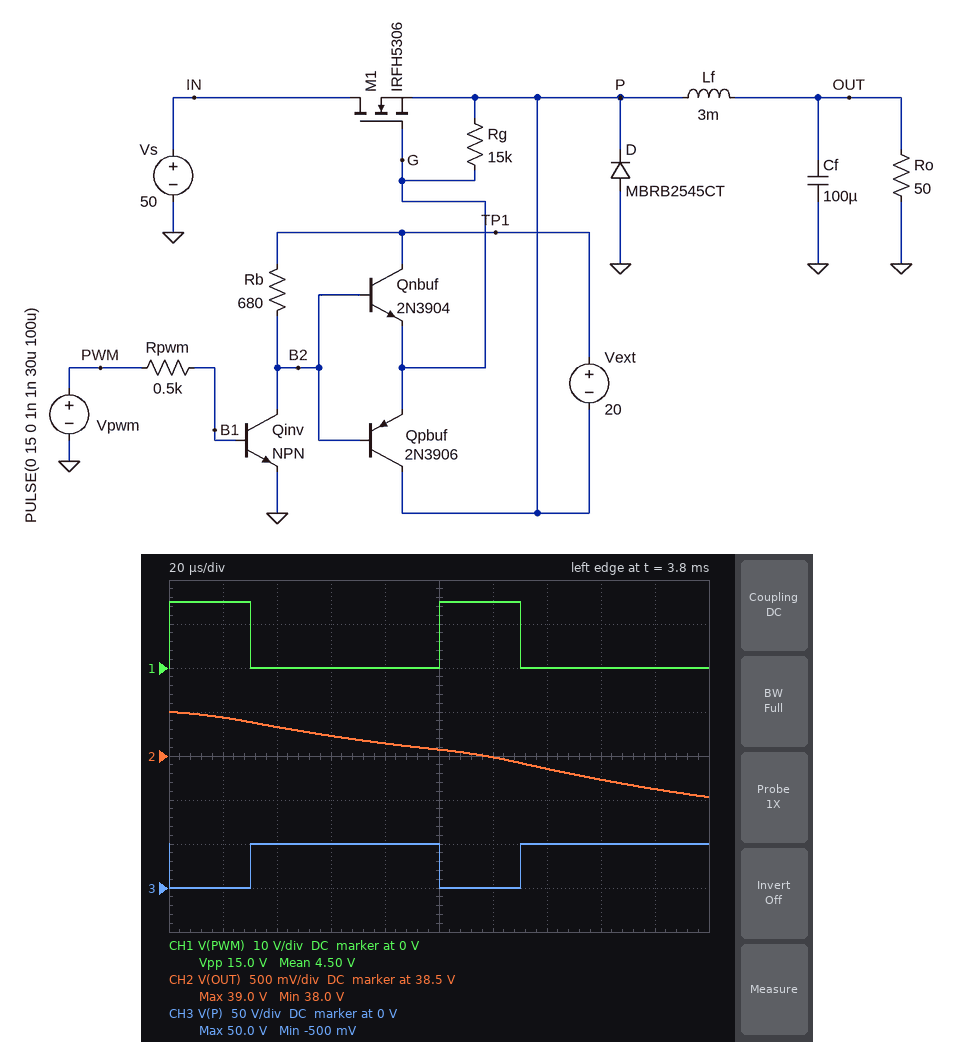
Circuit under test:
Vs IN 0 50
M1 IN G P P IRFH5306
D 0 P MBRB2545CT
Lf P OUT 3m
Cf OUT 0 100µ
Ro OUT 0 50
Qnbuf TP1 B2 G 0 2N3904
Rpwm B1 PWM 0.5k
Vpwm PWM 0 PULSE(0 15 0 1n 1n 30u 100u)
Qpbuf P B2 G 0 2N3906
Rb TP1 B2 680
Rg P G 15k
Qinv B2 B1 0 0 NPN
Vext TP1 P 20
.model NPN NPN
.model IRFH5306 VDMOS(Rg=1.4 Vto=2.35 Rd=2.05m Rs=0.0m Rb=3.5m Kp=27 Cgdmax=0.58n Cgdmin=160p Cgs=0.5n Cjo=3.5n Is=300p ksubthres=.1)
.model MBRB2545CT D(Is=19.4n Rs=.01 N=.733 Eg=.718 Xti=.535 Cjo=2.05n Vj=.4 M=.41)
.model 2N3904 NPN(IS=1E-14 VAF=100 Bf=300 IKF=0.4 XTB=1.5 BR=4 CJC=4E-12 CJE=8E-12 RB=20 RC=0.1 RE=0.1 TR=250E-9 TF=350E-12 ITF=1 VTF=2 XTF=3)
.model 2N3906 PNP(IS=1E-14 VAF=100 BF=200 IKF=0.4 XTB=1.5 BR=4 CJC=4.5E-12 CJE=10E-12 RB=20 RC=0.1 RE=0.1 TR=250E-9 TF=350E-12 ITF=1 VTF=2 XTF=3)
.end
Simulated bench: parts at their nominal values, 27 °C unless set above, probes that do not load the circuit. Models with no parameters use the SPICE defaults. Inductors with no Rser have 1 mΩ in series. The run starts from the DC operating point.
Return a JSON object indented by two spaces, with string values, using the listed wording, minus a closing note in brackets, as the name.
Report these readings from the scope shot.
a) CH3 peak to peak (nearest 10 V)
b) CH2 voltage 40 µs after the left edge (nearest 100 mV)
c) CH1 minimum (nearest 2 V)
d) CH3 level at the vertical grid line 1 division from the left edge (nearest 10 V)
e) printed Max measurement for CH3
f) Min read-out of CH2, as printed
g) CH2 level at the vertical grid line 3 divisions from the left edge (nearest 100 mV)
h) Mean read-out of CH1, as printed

{
  "CH3 peak to peak": "50 V",
  "CH2 voltage 40 µs after the left edge": "38.8 V",
  "CH1 minimum": "0 V",
  "CH3 level at the vertical grid line 1 division from the left edge": "0 V",
  "printed Max measurement for CH3": "50.0 V",
  "Min read-out of CH2, as printed": "38.0 V",
  "CH2 level at the vertical grid line 3 divisions from the left edge": "38.7 V",
  "Mean read-out of CH1, as printed": "4.50 V"
}
